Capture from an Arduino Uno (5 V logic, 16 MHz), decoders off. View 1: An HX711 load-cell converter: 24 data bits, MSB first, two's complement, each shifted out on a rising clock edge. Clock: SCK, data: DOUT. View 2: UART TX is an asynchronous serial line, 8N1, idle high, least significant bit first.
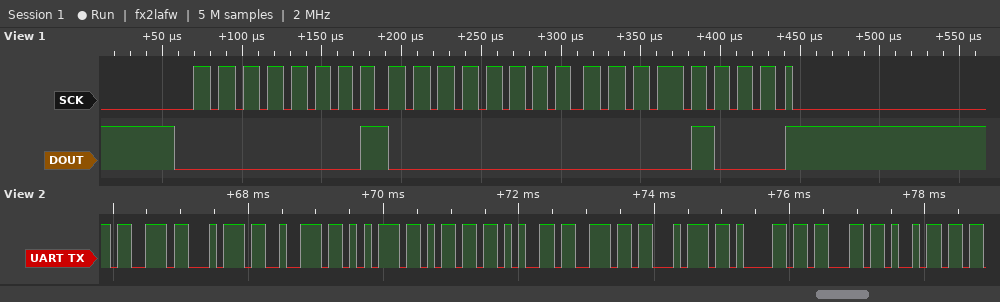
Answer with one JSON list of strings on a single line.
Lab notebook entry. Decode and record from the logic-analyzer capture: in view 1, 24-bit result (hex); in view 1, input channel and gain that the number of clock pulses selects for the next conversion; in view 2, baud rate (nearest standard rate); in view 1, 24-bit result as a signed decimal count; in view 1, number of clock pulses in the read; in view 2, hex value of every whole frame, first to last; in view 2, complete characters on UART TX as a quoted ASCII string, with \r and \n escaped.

["0x010008", "channel A, gain 128", "9600 baud", "65544", "25", "0x73 0x74 0x72 0x75 0x6D 0x65 0x6E 0x74 0x61 0x63 0x69", "\"strumentaci\""]
